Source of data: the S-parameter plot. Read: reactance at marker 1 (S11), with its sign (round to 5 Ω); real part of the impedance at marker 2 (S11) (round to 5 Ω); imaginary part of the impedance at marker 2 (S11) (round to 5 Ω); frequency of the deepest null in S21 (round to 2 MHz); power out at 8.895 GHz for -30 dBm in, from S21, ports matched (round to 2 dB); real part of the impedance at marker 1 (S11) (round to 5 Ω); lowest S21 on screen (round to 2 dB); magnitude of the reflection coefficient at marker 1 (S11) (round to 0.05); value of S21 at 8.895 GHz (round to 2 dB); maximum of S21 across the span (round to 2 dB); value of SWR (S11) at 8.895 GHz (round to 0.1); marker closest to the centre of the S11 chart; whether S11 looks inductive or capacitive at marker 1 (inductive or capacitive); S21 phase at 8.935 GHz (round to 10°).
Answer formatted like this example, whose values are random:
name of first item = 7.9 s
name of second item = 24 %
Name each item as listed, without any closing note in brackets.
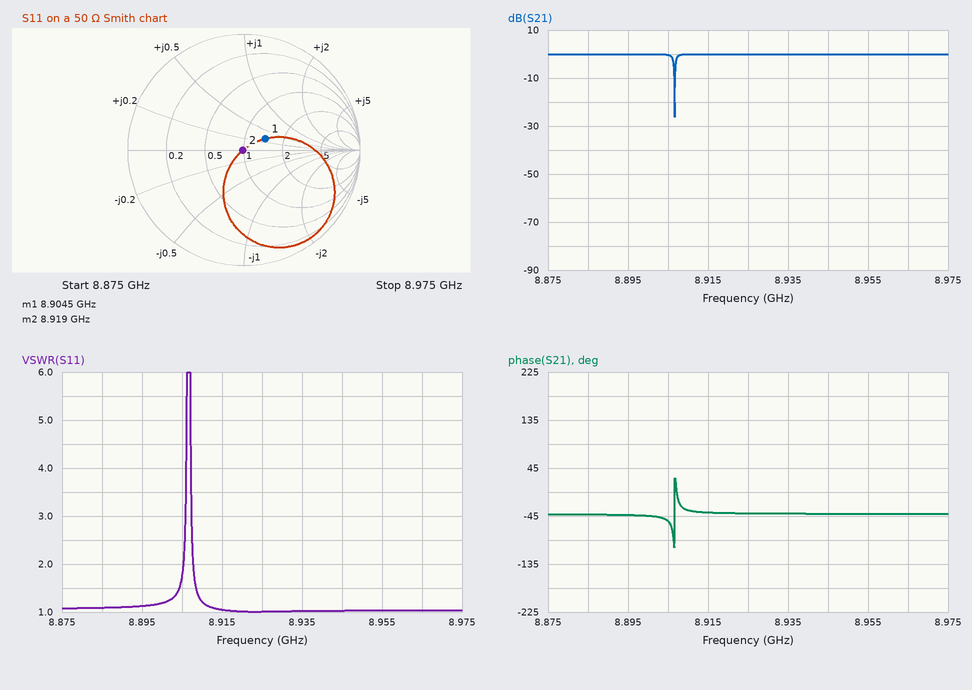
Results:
reactance at marker 1 (S11), with its sign = +15 Ω
real part of the impedance at marker 2 (S11) = 50 Ω
imaginary part of the impedance at marker 2 (S11) = 0 Ω
frequency of the deepest null in S21 = 8.906 GHz
power out at 8.895 GHz for -30 dBm in, from S21, ports matched = -30 dBm
real part of the impedance at marker 1 (S11) = 70 Ω
lowest S21 on screen = -26 dB
magnitude of the reflection coefficient at marker 1 (S11) = 0.20
value of S21 at 8.895 GHz = 0 dB
maximum of S21 across the span = 0 dB
value of SWR (S11) at 8.895 GHz = 1.1
marker closest to the centre of the S11 chart = marker 2
whether S11 looks inductive or capacitive at marker 1 = inductive
S21 phase at 8.935 GHz = -40°
